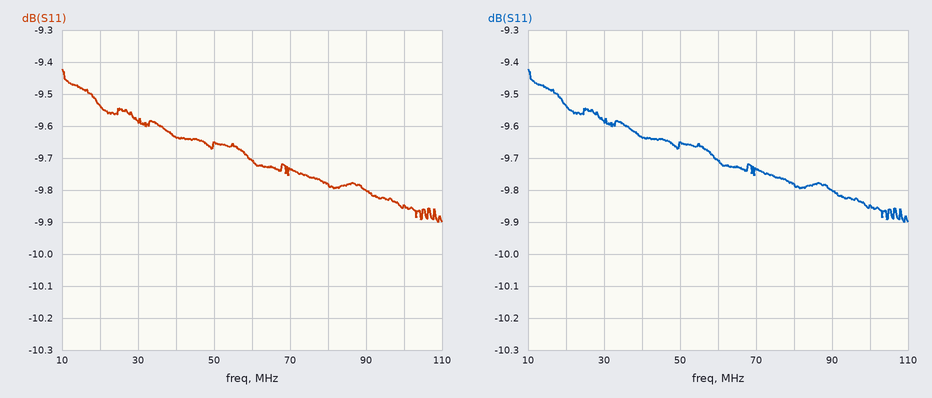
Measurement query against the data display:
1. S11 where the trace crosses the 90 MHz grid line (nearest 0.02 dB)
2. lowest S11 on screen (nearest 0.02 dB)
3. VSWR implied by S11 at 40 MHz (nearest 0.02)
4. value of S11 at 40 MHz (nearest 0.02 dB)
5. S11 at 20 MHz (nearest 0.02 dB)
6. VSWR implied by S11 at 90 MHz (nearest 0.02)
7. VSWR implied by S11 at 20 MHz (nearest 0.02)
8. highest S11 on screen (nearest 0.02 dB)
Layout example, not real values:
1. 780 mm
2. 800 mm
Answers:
1. -9.80 dB
2. -9.90 dB
3. 1.98
4. -9.64 dB
5. -9.54 dB
6. 1.96
7. 2.00
8. -9.42 dB
